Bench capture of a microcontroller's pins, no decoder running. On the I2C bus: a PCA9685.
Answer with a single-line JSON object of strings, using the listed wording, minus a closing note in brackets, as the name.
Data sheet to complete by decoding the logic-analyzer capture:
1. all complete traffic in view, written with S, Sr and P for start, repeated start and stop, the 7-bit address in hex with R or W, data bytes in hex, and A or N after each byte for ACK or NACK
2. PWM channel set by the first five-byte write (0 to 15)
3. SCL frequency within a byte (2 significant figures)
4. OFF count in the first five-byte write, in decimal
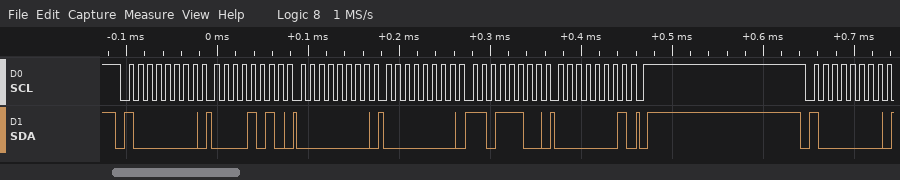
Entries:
{"all complete traffic in view, written with S, Sr and P for start, repeated start and stop, the 7-bit address in hex with R or W, data bytes in hex, and A or N after each byte for ACK or NACK": "S 40W A 0A A 00 A 00 A DC A 01 A P S 40W A", "PWM channel set by the first five-byte write": "1", "SCL frequency within a byte": "100 kHz", "OFF count in the first five-byte write, in decimal": "476"}
